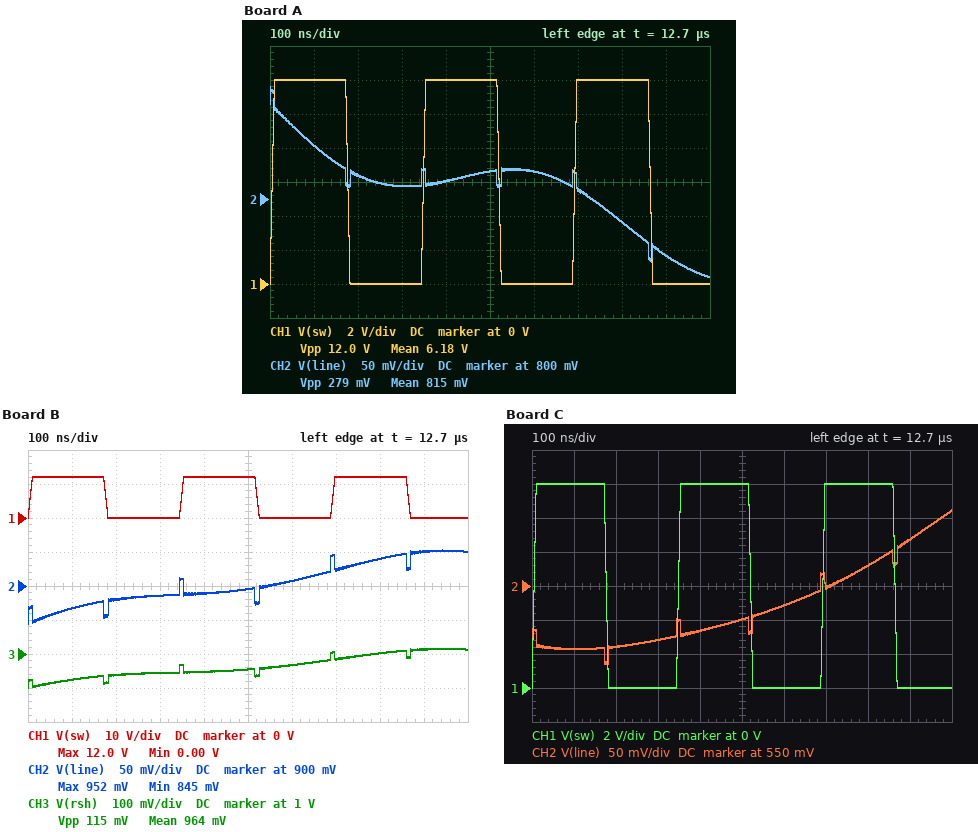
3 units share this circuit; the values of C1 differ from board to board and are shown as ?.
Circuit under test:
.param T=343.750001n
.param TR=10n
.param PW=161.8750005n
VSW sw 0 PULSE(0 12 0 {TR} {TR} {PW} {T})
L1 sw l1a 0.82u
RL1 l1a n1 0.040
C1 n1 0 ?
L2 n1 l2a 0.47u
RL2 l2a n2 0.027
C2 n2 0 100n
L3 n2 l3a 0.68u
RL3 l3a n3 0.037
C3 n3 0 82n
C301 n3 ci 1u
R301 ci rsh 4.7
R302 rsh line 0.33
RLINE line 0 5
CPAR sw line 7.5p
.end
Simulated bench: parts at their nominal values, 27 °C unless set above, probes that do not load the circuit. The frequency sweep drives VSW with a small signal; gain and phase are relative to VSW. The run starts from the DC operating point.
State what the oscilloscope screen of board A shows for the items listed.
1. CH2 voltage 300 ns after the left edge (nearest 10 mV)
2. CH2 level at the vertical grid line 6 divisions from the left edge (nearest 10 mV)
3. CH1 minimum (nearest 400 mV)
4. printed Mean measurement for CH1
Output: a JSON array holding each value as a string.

["820 mV", "840 mV", "0 V", "6.18 V"]
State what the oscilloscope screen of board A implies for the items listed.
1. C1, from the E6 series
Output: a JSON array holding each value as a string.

["100 nF"]
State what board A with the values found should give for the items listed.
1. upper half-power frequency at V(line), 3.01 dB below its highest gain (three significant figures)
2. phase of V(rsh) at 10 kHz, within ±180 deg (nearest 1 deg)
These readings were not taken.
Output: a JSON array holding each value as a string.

["328 kHz", "57 deg"]
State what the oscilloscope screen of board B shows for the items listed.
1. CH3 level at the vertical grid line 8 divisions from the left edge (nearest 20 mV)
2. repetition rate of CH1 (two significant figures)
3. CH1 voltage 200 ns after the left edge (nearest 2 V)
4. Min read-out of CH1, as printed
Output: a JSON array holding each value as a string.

["1.00 V", "2.9 MHz", "0 V", "0.00 V"]
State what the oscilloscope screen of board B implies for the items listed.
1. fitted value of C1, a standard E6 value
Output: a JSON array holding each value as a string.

["220 nF"]
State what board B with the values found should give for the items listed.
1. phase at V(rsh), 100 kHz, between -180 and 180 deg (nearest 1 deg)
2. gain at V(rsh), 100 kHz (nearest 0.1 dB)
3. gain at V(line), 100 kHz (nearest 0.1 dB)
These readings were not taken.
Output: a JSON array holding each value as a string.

["0 deg", "-3.9 dB", "-4.4 dB"]
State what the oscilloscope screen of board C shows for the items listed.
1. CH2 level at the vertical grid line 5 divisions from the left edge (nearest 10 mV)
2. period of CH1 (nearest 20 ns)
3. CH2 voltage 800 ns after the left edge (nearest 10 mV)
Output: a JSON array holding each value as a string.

["500 mV", "340 ns", "580 mV"]
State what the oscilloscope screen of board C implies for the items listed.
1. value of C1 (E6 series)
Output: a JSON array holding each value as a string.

["330 nF"]
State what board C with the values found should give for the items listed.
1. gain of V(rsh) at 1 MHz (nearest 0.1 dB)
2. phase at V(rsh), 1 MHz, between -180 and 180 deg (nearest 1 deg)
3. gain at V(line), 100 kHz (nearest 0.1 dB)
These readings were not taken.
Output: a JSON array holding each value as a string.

["-21.2 dB", "2 deg", "-4.1 dB"]
